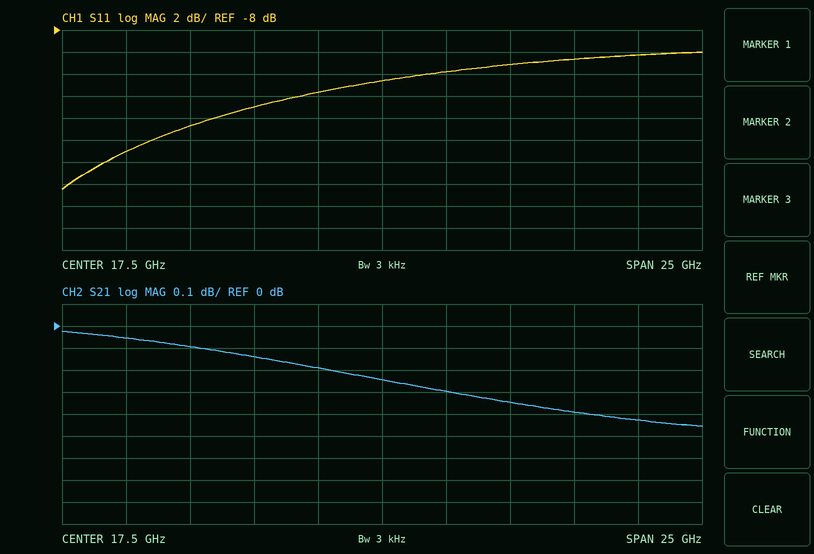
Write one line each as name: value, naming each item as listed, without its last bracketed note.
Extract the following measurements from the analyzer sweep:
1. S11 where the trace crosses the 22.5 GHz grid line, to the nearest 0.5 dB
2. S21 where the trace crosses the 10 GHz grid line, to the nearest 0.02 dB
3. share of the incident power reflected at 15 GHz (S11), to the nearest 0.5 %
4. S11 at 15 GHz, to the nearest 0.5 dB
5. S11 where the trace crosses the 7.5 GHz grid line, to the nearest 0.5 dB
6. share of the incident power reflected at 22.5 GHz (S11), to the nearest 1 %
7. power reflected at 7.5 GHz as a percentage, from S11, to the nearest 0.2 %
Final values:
S11 where the trace crosses the 22.5 GHz grid line, to the nearest 0.5 dB: -11.0 dB
S21 where the trace crosses the 10 GHz grid line, to the nearest 0.02 dB: -0.10 dB
share of the incident power reflected at 15 GHz (S11), to the nearest 0.5 %: 4.5 %
S11 at 15 GHz, to the nearest 0.5 dB: -13.5 dB
S11 where the trace crosses the 7.5 GHz grid line, to the nearest 0.5 dB: -19.0 dB
share of the incident power reflected at 22.5 GHz (S11), to the nearest 1 %: 8 %
power reflected at 7.5 GHz as a percentage, from S11, to the nearest 0.2 %: 1.2 %
